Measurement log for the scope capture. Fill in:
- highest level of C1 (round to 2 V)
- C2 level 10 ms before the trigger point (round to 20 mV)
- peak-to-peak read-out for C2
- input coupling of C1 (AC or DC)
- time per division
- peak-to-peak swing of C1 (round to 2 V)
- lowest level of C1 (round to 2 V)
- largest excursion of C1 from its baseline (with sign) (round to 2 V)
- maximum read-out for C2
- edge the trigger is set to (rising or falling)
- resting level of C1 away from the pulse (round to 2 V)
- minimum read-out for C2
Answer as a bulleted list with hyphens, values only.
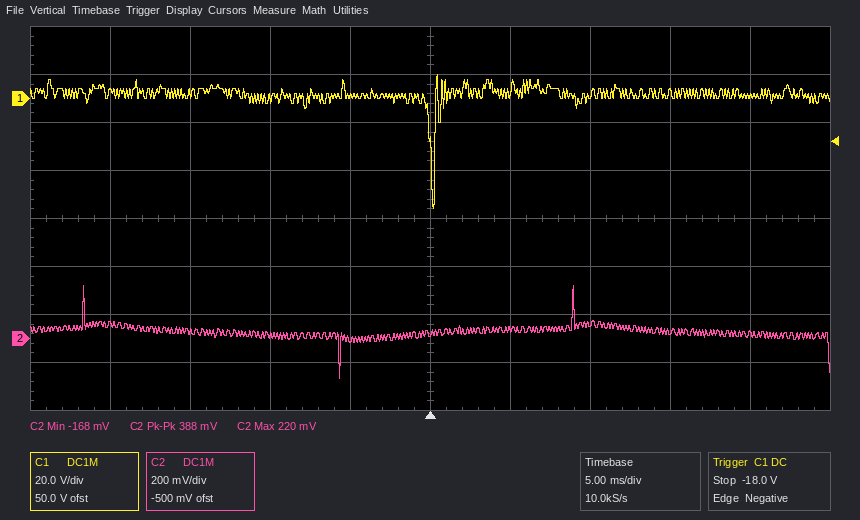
- 10 V
- 20 mV
- 388 mV
- DC
- 5 ms
- 56 V
- -46 V
- -48 V
- 220 mV
- falling
- 2 V
- -168 mV
